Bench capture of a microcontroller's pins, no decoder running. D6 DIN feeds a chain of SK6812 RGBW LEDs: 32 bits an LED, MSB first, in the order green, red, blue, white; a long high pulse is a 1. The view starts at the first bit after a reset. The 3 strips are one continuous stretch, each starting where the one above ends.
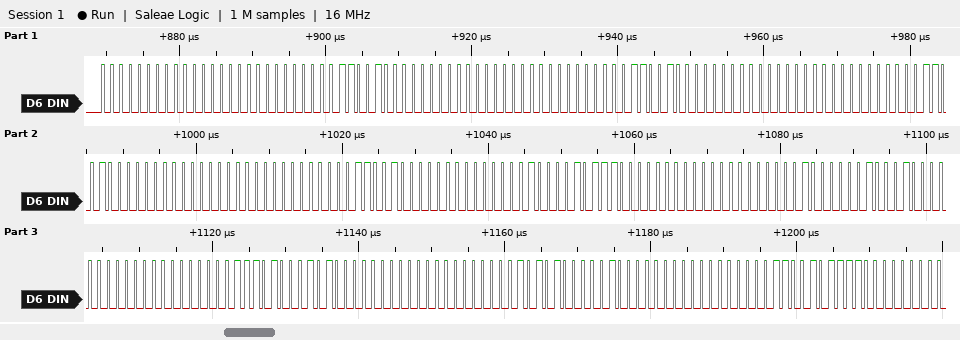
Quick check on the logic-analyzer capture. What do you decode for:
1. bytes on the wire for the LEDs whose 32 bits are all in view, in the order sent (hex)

00 00 00 32 00 00 00 32 00 00 00 32 00 00 00 32 00 04 2E 00 00 10 22 00 00 1D 14 00 00 2A 08 00
